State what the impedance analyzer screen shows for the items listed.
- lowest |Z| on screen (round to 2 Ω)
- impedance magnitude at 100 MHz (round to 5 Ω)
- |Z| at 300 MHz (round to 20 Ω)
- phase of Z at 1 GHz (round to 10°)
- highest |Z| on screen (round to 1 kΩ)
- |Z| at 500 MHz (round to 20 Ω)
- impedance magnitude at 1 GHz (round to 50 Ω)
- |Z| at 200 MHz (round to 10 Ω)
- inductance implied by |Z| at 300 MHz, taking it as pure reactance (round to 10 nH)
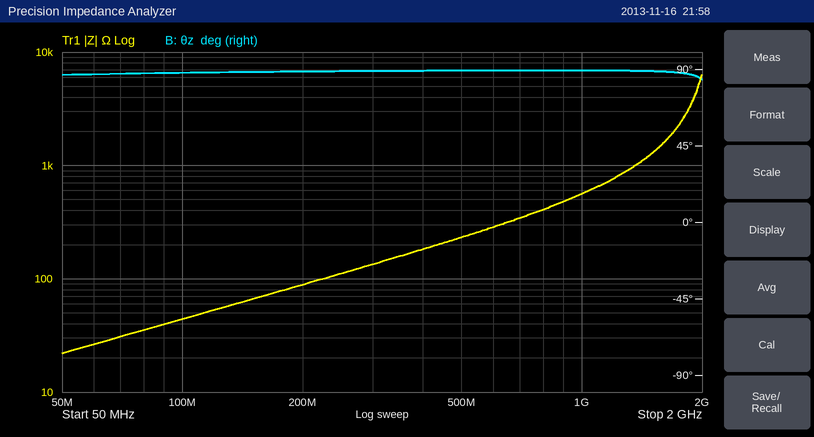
22 Ω
45 Ω
140 Ω
90°
6 kΩ
240 Ω
550 Ω
90 Ω
70 nH
